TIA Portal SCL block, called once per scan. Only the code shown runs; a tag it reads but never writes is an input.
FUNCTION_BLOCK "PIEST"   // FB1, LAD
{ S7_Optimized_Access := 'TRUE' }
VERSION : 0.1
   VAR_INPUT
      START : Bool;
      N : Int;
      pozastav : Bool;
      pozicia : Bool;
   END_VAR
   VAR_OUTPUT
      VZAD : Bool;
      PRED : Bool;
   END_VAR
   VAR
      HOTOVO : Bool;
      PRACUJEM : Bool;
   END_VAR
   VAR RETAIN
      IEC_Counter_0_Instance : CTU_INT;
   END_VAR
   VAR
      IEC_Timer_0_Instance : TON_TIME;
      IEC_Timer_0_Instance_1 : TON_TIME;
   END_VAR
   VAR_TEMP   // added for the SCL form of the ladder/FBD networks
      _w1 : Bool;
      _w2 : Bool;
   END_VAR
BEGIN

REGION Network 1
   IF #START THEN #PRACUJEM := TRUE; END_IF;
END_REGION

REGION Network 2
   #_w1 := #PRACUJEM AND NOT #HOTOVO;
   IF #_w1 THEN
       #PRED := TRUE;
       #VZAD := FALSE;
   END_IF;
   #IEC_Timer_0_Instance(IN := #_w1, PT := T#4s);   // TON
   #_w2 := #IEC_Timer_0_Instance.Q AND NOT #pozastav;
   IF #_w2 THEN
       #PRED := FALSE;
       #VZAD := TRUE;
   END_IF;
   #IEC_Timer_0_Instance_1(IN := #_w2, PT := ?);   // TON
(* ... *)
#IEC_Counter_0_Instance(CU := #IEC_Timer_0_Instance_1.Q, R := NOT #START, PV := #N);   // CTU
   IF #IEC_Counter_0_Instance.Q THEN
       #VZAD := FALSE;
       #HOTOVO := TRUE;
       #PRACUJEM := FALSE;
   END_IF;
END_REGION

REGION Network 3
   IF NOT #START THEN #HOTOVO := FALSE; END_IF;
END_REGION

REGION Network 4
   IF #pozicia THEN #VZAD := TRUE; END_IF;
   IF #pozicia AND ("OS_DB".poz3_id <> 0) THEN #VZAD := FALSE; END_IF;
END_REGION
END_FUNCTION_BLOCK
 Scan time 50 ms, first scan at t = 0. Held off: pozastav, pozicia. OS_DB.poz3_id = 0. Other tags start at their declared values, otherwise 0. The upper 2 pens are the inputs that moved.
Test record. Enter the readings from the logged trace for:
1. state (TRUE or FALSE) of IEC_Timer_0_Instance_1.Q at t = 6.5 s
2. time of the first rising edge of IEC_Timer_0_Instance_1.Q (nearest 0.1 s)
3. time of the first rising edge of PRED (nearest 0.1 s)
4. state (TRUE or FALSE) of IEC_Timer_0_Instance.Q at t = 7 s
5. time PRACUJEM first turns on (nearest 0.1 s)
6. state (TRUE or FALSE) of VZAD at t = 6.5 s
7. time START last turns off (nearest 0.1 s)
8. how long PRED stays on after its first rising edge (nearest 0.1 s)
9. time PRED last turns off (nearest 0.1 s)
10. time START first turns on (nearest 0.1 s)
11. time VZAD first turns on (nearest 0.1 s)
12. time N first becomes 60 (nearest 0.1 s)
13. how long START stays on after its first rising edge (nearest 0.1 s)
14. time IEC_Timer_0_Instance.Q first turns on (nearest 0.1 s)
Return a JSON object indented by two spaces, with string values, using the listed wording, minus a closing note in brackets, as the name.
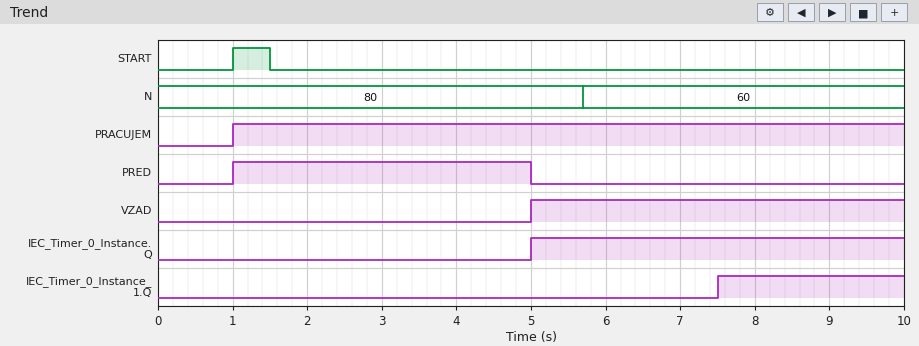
{
  "state (TRUE or FALSE) of IEC_Timer_0_Instance_1.Q at t = 6.5 s": "FALSE",
  "time of the first rising edge of IEC_Timer_0_Instance_1.Q": "7.5 s",
  "time of the first rising edge of PRED": "1.0 s",
  "state (TRUE or FALSE) of IEC_Timer_0_Instance.Q at t = 7 s": "TRUE",
  "time PRACUJEM first turns on": "1.0 s",
  "state (TRUE or FALSE) of VZAD at t = 6.5 s": "TRUE",
  "time START last turns off": "1.5 s",
  "how long PRED stays on after its first rising edge": "4.0 s",
  "time PRED last turns off": "5.0 s",
  "time START first turns on": "1.0 s",
  "time VZAD first turns on": "5.0 s",
  "time N first becomes 60": "5.7 s",
  "how long START stays on after its first rising edge": "0.5 s",
  "time IEC_Timer_0_Instance.Q first turns on": "5.0 s"
}
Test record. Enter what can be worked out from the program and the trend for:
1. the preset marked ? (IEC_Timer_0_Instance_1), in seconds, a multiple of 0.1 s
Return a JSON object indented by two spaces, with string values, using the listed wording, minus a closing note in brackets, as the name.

{
  "the preset marked ? (IEC_Timer_0_Instance_1), in seconds, a multiple of 0.1 s": "2.5 s"
}
